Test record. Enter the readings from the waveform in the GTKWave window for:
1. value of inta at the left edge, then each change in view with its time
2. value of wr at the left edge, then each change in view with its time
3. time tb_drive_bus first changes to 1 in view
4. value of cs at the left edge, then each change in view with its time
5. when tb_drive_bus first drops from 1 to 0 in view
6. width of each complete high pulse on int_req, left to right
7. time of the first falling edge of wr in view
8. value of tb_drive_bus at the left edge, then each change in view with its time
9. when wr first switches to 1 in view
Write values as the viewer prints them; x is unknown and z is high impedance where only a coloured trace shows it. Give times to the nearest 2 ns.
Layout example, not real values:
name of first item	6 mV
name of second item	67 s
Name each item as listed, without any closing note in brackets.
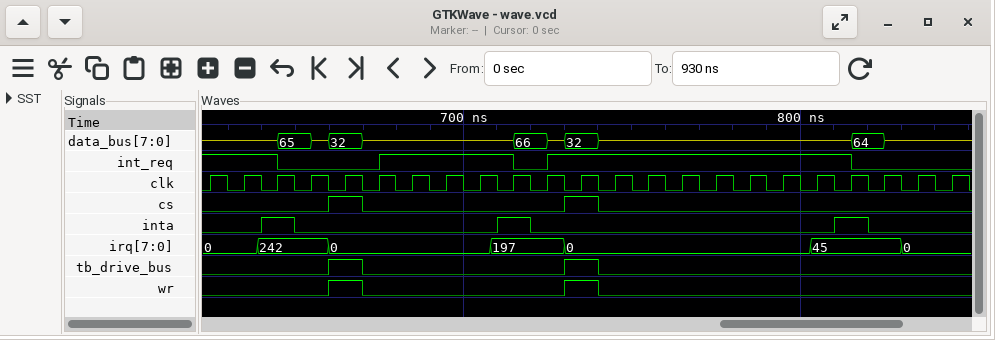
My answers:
value of inta at the left edge, then each change in view with its time	0, 1 at 640 ns, 0 at 650 ns, 1 at 710 ns, 0 at 720 ns, 1 at 810 ns, 0 at 820 ns
value of wr at the left edge, then each change in view with its time	0, 1 at 660 ns, 0 at 670 ns, 1 at 730 ns, 0 at 740 ns
time tb_drive_bus first changes to 1 in view	660 ns
value of cs at the left edge, then each change in view with its time	0, 1 at 660 ns, 0 at 670 ns, 1 at 730 ns, 0 at 740 ns
when tb_drive_bus first drops from 1 to 0 in view	670 ns
width of each complete high pulse on int_req, left to right	40 ns, 90 ns
time of the first falling edge of wr in view	670 ns
value of tb_drive_bus at the left edge, then each change in view with its time	0, 1 at 660 ns, 0 at 670 ns, 1 at 730 ns, 0 at 740 ns
when wr first switches to 1 in view	660 ns
